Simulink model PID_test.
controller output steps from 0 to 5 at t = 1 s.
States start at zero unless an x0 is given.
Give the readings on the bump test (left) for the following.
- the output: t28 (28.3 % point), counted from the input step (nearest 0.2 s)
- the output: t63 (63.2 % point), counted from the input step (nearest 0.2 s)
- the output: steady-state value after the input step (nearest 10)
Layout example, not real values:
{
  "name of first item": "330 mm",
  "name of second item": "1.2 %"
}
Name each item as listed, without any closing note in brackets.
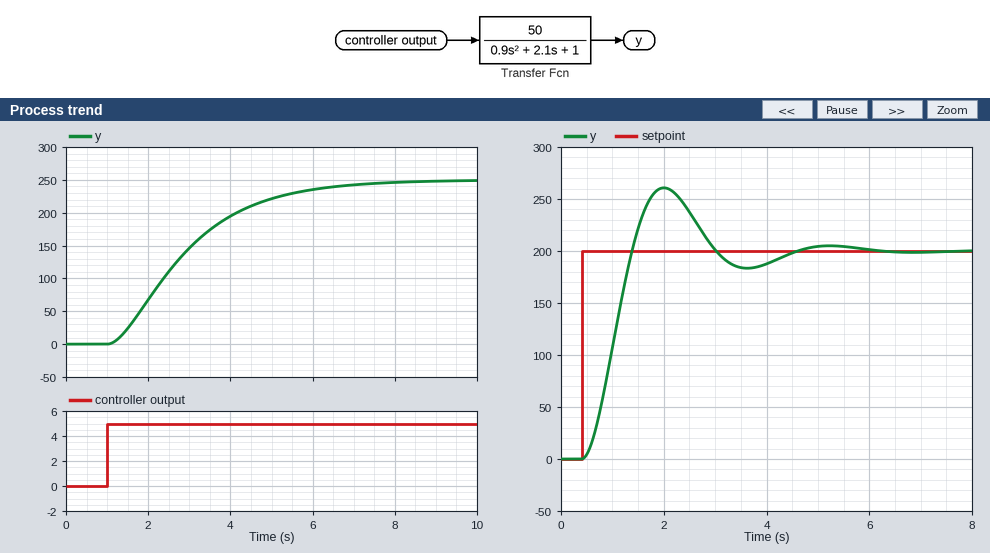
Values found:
{
  "the output: t28 (28.3 % point), counted from the input step": "1.0 s",
  "the output: t63 (63.2 % point), counted from the input step": "2.2 s",
  "the output: steady-state value after the input step": "250"
}
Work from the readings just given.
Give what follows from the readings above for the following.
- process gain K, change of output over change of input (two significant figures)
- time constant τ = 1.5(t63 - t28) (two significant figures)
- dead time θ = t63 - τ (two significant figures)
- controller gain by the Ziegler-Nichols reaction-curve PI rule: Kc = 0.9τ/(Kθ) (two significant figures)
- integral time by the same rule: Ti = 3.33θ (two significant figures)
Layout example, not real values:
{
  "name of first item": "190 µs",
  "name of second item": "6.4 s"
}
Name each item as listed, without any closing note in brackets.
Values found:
{
  "process gain K, change of output over change of input": "50",
  "time constant τ = 1.5(t63 - t28)": "1.8 s",
  "dead time θ = t63 - τ": "0.40 s",
  "controller gain by the Ziegler-Nichols reaction-curve PI rule: Kc = 0.9τ/(Kθ)": "0.081",
  "integral time by the same rule: Ti = 3.33θ": "1.3 s"
}
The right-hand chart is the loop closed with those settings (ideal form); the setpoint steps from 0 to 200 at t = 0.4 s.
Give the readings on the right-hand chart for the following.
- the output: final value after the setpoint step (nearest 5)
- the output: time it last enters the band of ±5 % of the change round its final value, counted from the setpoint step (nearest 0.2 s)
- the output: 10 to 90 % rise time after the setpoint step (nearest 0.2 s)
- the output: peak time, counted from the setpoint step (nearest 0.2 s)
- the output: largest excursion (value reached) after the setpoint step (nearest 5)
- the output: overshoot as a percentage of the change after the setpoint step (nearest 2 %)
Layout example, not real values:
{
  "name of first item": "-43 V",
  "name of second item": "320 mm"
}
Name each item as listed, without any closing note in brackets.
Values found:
{
  "the output: final value after the setpoint step": "200",
  "the output: time it last enters the band of ±5 % of the change round its final value, counted from the setpoint step": "3.8 s",
  "the output: 10 to 90 % rise time after the setpoint step": "0.6 s",
  "the output: peak time, counted from the setpoint step": "1.6 s",
  "the output: largest excursion (value reached) after the setpoint step": "260",
  "the output: overshoot as a percentage of the change after the setpoint step": "30 %"
}
